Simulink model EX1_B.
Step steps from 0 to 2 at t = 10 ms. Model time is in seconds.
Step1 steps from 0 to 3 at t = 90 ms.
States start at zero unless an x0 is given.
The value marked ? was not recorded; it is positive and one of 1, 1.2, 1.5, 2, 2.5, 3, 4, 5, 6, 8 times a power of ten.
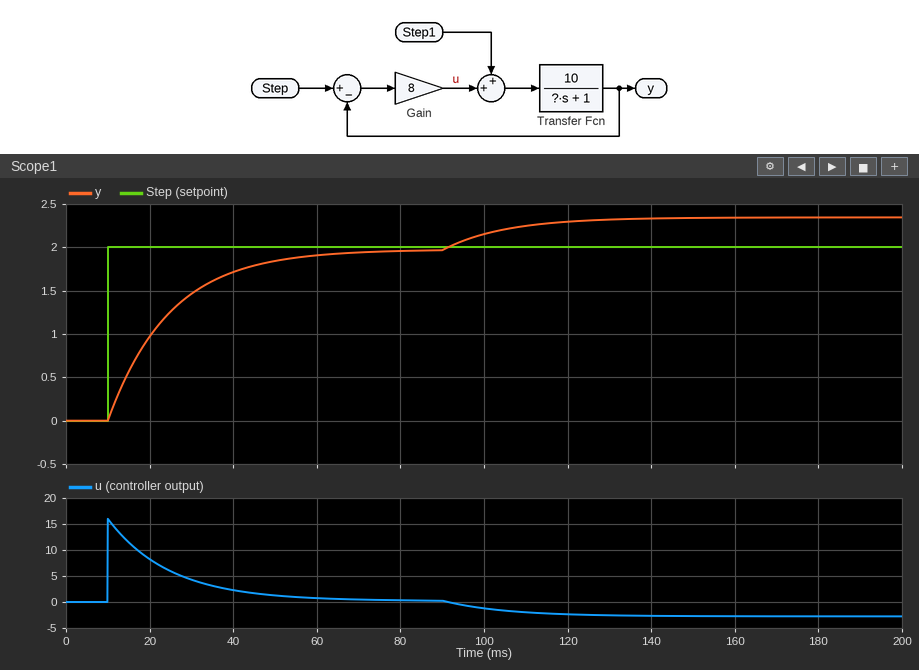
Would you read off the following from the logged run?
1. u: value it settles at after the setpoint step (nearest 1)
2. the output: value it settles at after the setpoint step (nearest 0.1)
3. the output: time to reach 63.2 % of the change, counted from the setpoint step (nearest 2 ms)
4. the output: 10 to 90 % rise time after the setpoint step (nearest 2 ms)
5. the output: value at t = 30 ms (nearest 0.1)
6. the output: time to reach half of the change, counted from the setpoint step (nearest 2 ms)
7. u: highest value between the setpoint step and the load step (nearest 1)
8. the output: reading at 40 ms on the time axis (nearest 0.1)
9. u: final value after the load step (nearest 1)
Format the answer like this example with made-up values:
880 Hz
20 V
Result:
0
2.0
14 ms
32 ms
1.5
10 ms
16
1.7
-3
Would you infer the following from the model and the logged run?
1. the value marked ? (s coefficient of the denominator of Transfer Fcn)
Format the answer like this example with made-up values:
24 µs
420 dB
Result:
1.2
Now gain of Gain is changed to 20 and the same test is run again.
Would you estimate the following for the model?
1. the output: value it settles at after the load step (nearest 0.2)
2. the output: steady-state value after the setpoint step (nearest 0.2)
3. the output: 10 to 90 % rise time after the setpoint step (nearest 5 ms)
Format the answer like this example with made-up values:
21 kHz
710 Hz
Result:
2.2
2.0
15 ms
